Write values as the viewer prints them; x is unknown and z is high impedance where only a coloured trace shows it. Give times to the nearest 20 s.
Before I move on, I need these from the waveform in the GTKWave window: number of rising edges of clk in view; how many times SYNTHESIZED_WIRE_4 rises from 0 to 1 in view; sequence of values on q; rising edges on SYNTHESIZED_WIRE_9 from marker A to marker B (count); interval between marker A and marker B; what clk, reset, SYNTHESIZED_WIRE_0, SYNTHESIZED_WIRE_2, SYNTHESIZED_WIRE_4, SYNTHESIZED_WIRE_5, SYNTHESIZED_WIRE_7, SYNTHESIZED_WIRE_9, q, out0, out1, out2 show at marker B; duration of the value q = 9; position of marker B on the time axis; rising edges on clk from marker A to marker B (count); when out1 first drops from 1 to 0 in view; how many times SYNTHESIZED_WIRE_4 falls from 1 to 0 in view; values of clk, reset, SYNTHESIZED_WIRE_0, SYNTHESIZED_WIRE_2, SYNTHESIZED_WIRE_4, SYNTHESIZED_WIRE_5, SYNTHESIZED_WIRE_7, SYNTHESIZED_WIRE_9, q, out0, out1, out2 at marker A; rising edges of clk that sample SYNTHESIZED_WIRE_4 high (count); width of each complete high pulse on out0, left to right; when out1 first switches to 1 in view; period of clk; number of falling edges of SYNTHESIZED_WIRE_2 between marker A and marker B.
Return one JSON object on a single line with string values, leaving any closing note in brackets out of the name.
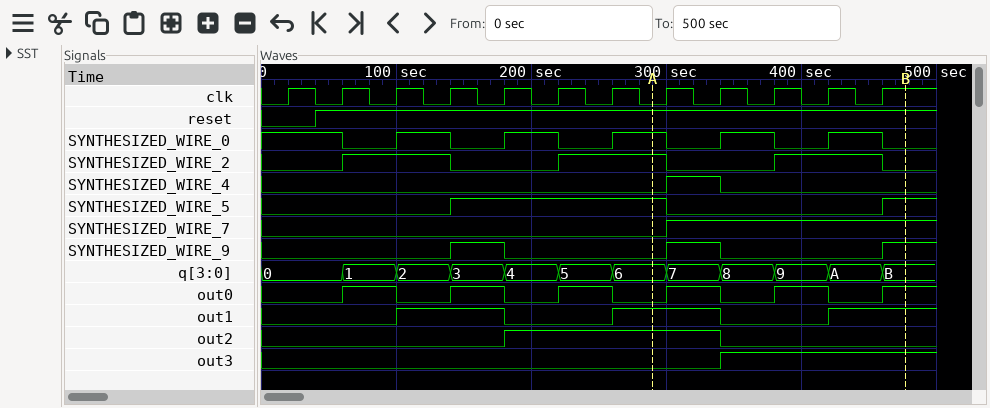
{"number of rising edges of clk in view": "12", "how many times SYNTHESIZED_WIRE_4 rises from 0 to 1 in view": "1", "sequence of values on q": "0, 1, 2, 3, 4, 5, 6, 7, 8, 9, A, B", "rising edges on SYNTHESIZED_WIRE_9 from marker A to marker B": "2", "interval between marker A and marker B": "180 s", "what clk, reset, SYNTHESIZED_WIRE_0, SYNTHESIZED_WIRE_2, SYNTHESIZED_WIRE_4, SYNTHESIZED_WIRE_5, SYNTHESIZED_WIRE_7, SYNTHESIZED_WIRE_9, q, out0, out1, out2 show at marker B": "clk=1, reset=1, SYNTHESIZED_WIRE_0=0, SYNTHESIZED_WIRE_2=0, SYNTHESIZED_WIRE_4=0, SYNTHESIZED_WIRE_5=1, SYNTHESIZED_WIRE_7=1, SYNTHESIZED_WIRE_9=1, q=B, out0=1, out1=1, out2=0", "duration of the value q = 9": "40 s", "position of marker B on the time axis": "480 s", "rising edges on clk from marker A to marker B": "5", "when out1 first drops from 1 to 0 in view": "180 s", "how many times SYNTHESIZED_WIRE_4 falls from 1 to 0 in view": "1", "values of clk, reset, SYNTHESIZED_WIRE_0, SYNTHESIZED_WIRE_2, SYNTHESIZED_WIRE_4, SYNTHESIZED_WIRE_5, SYNTHESIZED_WIRE_7, SYNTHESIZED_WIRE_9, q, out0, out1, out2 at marker A": "clk=0, reset=1, SYNTHESIZED_WIRE_0=1, SYNTHESIZED_WIRE_2=1, SYNTHESIZED_WIRE_4=0, SYNTHESIZED_WIRE_5=1, SYNTHESIZED_WIRE_7=0, SYNTHESIZED_WIRE_9=0, q=6, out0=0, out1=1, out2=1", "rising edges of clk that sample SYNTHESIZED_WIRE_4 high": "1", "width of each complete high pulse on out0, left to right": "40 s, 40 s, 40 s, 40 s, 40 s", "when out1 first switches to 1 in view": "100 s", "period of clk": "40 s", "number of falling edges of SYNTHESIZED_WIRE_2 between marker A and marker B": "2"}
